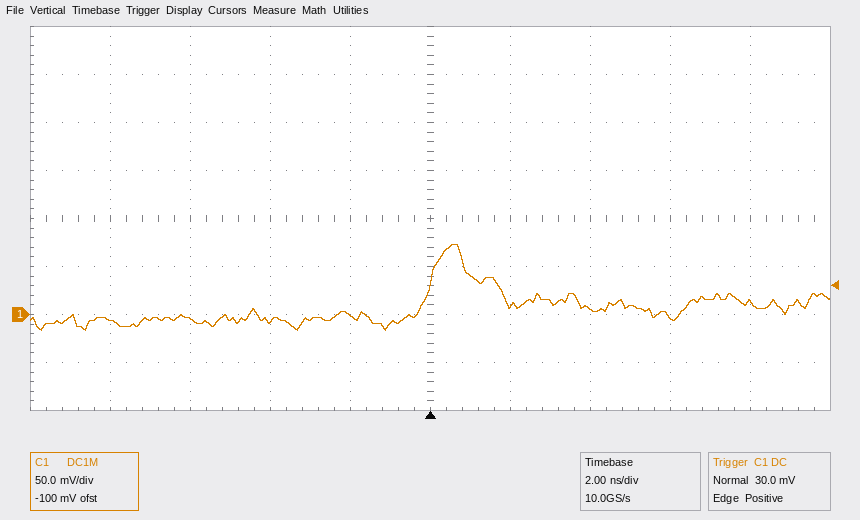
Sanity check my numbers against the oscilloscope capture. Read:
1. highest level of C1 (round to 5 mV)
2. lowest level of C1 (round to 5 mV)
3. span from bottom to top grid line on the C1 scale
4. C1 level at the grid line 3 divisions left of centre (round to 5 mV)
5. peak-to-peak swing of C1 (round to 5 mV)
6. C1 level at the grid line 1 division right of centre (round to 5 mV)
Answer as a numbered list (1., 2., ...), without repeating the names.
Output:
1. 75 mV
2. -15 mV
3. 400 mV
4. -5 mV
5. 90 mV
6. 10 mV
